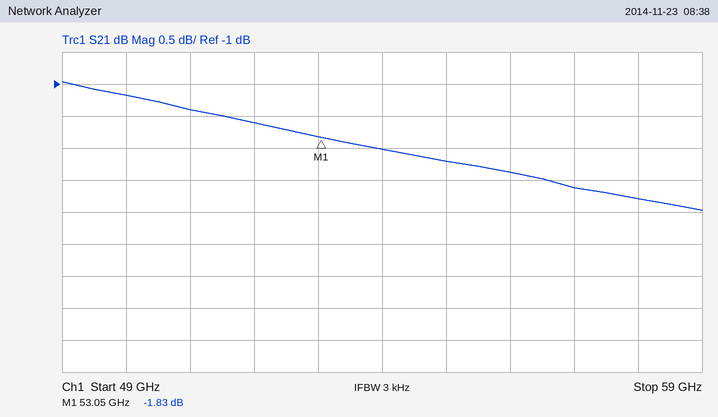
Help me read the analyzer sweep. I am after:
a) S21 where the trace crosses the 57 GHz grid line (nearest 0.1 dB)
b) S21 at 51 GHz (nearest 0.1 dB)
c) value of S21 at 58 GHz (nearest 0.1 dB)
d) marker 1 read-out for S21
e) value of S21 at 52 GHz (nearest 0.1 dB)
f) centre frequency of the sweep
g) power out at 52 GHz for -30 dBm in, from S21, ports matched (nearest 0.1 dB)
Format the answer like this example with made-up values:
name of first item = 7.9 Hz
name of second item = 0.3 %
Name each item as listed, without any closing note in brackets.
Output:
S21 where the trace crosses the 57 GHz grid line = -2.6 dB
S21 at 51 GHz = -1.4 dB
value of S21 at 58 GHz = -2.8 dB
marker 1 read-out for S21 = -1.83 dB
value of S21 at 52 GHz = -1.6 dB
centre frequency of the sweep = 54 GHz
power out at 52 GHz for -30 dBm in, from S21, ports matched = -31.6 dBm
